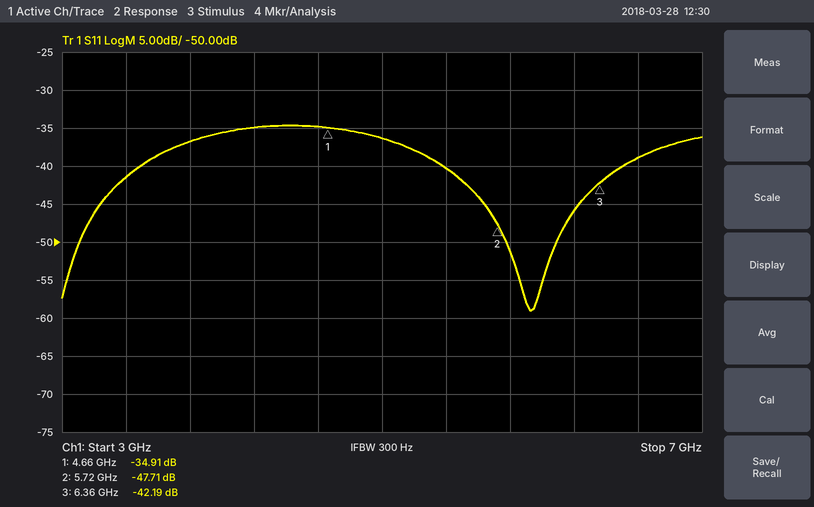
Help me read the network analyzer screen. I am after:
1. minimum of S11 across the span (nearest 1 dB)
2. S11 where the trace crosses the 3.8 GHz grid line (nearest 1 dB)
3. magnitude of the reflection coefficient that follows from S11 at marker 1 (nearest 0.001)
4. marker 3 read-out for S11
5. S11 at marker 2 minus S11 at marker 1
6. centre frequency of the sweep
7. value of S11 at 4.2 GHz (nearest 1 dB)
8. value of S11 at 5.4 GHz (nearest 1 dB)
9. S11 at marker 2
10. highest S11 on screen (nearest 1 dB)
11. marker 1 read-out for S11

-59 dB
-37 dB
0.018
-42.19 dB
-12.80 dB
5 GHz
-35 dB
-40 dB
-47.71 dB
-35 dB
-34.91 dB
